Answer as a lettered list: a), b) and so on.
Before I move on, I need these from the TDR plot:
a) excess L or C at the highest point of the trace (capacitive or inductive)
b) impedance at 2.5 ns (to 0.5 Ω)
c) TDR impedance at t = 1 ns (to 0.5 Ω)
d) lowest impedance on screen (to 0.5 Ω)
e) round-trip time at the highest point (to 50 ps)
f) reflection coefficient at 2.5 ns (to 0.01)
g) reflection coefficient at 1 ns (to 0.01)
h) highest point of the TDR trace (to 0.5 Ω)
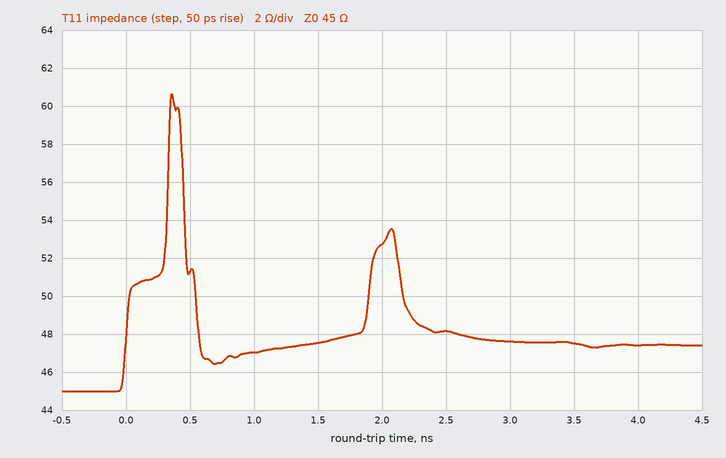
a) inductive
b) 48.0 Ω
c) 47.0 Ω
d) 45.0 Ω
e) 350 ps
f) +0.03
g) +0.02
h) 60.5 Ω
